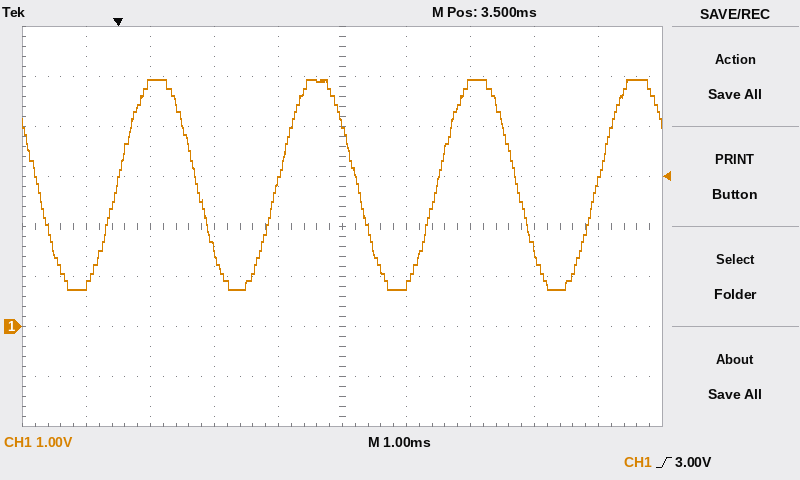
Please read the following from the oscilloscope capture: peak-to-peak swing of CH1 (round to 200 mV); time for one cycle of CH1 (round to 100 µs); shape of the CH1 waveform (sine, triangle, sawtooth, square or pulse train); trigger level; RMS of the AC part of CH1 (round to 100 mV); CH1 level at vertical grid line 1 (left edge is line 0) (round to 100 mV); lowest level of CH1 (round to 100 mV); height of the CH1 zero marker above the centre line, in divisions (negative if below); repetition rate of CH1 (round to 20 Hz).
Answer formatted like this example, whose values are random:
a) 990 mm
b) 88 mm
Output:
a) 4.2 V
b) 2.5 ms
c) sine
d) 3.00 V
e) 1.5 V
f) 800 mV
g) 700 mV
h) -2.0 div
i) 400 Hz
